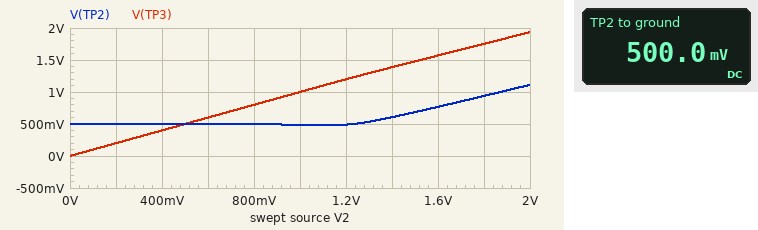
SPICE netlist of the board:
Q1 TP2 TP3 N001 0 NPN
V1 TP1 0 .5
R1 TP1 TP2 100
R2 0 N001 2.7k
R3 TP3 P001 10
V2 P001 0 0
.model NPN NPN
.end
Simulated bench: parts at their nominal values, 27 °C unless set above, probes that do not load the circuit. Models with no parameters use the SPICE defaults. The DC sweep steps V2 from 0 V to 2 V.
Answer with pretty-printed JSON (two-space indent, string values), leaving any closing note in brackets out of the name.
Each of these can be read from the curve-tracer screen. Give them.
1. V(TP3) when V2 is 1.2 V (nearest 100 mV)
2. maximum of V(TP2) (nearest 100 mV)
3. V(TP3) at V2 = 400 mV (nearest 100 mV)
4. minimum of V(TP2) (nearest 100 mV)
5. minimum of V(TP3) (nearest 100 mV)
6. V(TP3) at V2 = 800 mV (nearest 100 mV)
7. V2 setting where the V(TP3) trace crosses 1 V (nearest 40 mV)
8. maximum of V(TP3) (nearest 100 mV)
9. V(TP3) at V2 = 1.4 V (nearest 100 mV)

{
  "V(TP3) when V2 is 1.2 V": "1.2 V",
  "maximum of V(TP2)": "1.1 V",
  "V(TP3) at V2 = 400 mV": "400 mV",
  "minimum of V(TP2)": "500 mV",
  "minimum of V(TP3)": "0 V",
  "V(TP3) at V2 = 800 mV": "800 mV",
  "V2 setting where the V(TP3) trace crosses 1 V": "1.00 V",
  "maximum of V(TP3)": "1.9 V",
  "V(TP3) at V2 = 1.4 V": "1.4 V"
}
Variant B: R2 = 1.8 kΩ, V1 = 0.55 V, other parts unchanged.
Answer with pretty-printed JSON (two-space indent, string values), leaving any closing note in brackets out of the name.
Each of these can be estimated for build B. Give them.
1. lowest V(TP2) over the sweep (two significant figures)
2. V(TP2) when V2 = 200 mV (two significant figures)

{
  "lowest V(TP2) over the sweep": "530 mV",
  "V(TP2) when V2 = 200 mV": "550 mV"
}
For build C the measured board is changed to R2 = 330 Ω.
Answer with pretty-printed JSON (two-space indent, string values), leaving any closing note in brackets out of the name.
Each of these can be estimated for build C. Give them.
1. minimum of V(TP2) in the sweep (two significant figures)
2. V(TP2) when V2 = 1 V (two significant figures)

{
  "minimum of V(TP2) in the sweep": "410 mV",
  "V(TP2) when V2 = 1 V": "430 mV"
}
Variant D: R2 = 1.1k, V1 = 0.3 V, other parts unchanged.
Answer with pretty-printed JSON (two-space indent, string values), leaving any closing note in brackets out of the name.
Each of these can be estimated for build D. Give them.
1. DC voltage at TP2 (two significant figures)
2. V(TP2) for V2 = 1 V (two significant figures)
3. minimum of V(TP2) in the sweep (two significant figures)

{
  "DC voltage at TP2": "300 mV",
  "V(TP2) for V2 = 1 V": "290 mV",
  "minimum of V(TP2) in the sweep": "280 mV"
}
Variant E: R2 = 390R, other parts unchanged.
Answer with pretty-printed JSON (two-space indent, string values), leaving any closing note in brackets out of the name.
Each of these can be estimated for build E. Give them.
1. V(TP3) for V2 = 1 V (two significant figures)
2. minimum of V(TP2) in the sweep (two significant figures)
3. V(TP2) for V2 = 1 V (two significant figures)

{
  "V(TP3) for V2 = 1 V": "1.0 V",
  "minimum of V(TP2) in the sweep": "420 mV",
  "V(TP2) for V2 = 1 V": "440 mV"
}
